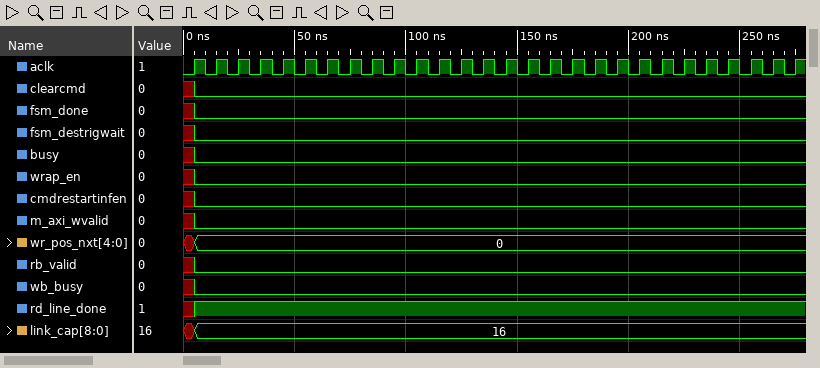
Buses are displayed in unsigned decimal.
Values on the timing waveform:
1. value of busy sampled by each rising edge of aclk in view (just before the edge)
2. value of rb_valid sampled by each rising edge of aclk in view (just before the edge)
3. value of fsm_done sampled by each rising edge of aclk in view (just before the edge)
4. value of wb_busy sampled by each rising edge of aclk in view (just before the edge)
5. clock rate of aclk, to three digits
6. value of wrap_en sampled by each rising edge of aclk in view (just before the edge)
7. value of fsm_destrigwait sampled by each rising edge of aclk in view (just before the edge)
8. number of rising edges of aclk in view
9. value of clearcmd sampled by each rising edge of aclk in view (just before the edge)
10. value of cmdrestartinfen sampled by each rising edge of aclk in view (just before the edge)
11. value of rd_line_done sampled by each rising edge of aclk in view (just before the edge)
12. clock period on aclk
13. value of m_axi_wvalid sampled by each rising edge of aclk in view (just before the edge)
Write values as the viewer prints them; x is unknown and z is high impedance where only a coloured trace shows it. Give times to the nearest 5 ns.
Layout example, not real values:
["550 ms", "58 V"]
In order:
["x 0 0 0 0 0 0 0 0 0 0 0 0 0 0 0 0 0 0 0 0 0 0 0 0 0 0 0", "x 0 0 0 0 0 0 0 0 0 0 0 0 0 0 0 0 0 0 0 0 0 0 0 0 0 0 0", "x 0 0 0 0 0 0 0 0 0 0 0 0 0 0 0 0 0 0 0 0 0 0 0 0 0 0 0", "x 0 0 0 0 0 0 0 0 0 0 0 0 0 0 0 0 0 0 0 0 0 0 0 0 0 0 0", "100 MHz", "x 0 0 0 0 0 0 0 0 0 0 0 0 0 0 0 0 0 0 0 0 0 0 0 0 0 0 0", "x 0 0 0 0 0 0 0 0 0 0 0 0 0 0 0 0 0 0 0 0 0 0 0 0 0 0 0", "28", "x 0 0 0 0 0 0 0 0 0 0 0 0 0 0 0 0 0 0 0 0 0 0 0 0 0 0 0", "x 0 0 0 0 0 0 0 0 0 0 0 0 0 0 0 0 0 0 0 0 0 0 0 0 0 0 0", "x 1 1 1 1 1 1 1 1 1 1 1 1 1 1 1 1 1 1 1 1 1 1 1 1 1 1 1", "10 ns", "x 0 0 0 0 0 0 0 0 0 0 0 0 0 0 0 0 0 0 0 0 0 0 0 0 0 0 0"]
